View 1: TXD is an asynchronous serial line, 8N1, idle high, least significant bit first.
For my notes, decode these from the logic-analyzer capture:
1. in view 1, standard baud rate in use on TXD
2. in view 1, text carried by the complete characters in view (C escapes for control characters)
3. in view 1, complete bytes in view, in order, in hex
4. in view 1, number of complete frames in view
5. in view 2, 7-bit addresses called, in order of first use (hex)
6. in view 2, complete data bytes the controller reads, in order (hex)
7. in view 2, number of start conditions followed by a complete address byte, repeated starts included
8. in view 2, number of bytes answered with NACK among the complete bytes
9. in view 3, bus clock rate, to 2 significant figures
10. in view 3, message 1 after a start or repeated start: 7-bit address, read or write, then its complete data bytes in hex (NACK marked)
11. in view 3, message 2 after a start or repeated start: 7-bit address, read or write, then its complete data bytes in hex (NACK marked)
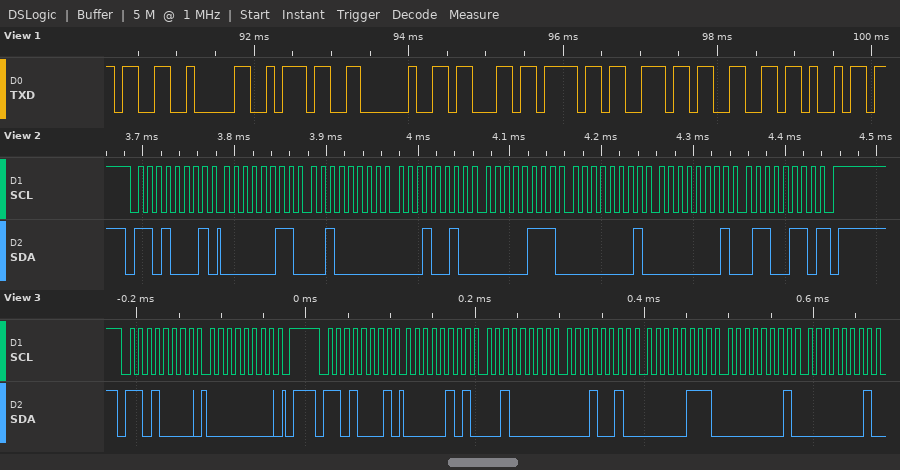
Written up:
9600 baud
"307 confi"
0x33 0x30 0x37 0x20 0x63 0x6F 0x6E 0x66 0x69
9
0x68
03 20 12 07 01 01 66
1
1
100 kHz
0x68 write: 00
0x68 read: 05 20 12 07 01 01
